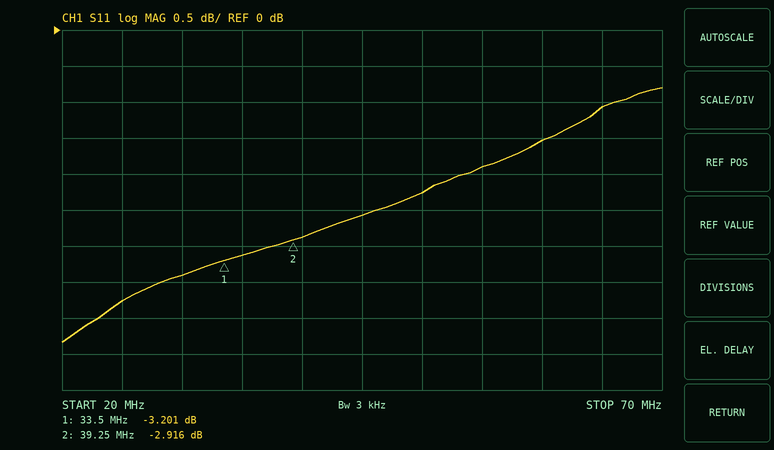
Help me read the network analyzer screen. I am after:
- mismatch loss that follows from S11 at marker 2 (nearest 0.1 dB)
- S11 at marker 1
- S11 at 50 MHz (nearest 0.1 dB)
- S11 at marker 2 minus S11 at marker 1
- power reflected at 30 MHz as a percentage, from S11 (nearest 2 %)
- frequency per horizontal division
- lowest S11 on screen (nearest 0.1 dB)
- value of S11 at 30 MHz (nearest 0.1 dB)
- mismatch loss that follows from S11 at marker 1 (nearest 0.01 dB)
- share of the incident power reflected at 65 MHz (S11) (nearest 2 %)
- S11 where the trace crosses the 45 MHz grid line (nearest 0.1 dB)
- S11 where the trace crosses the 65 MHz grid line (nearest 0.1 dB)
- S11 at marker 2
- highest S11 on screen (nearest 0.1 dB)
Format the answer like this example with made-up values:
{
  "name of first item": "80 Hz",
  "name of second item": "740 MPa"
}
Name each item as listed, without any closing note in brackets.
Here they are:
{
  "mismatch loss that follows from S11 at marker 2": "3.1 dB",
  "S11 at marker 1": "-3.201 dB",
  "S11 at 50 MHz": "-2.3 dB",
  "S11 at marker 2 minus S11 at marker 1": "0.285 dB",
  "power reflected at 30 MHz as a percentage, from S11": "46 %",
  "frequency per horizontal division": "5 MHz",
  "lowest S11 on screen": "-4.3 dB",
  "value of S11 at 30 MHz": "-3.4 dB",
  "mismatch loss that follows from S11 at marker 1": "2.83 dB",
  "share of the incident power reflected at 65 MHz (S11)": "78 %",
  "S11 where the trace crosses the 45 MHz grid line": "-2.6 dB",
  "S11 where the trace crosses the 65 MHz grid line": "-1.1 dB",
  "S11 at marker 2": "-2.916 dB",
  "highest S11 on screen": "-0.8 dB"
}
